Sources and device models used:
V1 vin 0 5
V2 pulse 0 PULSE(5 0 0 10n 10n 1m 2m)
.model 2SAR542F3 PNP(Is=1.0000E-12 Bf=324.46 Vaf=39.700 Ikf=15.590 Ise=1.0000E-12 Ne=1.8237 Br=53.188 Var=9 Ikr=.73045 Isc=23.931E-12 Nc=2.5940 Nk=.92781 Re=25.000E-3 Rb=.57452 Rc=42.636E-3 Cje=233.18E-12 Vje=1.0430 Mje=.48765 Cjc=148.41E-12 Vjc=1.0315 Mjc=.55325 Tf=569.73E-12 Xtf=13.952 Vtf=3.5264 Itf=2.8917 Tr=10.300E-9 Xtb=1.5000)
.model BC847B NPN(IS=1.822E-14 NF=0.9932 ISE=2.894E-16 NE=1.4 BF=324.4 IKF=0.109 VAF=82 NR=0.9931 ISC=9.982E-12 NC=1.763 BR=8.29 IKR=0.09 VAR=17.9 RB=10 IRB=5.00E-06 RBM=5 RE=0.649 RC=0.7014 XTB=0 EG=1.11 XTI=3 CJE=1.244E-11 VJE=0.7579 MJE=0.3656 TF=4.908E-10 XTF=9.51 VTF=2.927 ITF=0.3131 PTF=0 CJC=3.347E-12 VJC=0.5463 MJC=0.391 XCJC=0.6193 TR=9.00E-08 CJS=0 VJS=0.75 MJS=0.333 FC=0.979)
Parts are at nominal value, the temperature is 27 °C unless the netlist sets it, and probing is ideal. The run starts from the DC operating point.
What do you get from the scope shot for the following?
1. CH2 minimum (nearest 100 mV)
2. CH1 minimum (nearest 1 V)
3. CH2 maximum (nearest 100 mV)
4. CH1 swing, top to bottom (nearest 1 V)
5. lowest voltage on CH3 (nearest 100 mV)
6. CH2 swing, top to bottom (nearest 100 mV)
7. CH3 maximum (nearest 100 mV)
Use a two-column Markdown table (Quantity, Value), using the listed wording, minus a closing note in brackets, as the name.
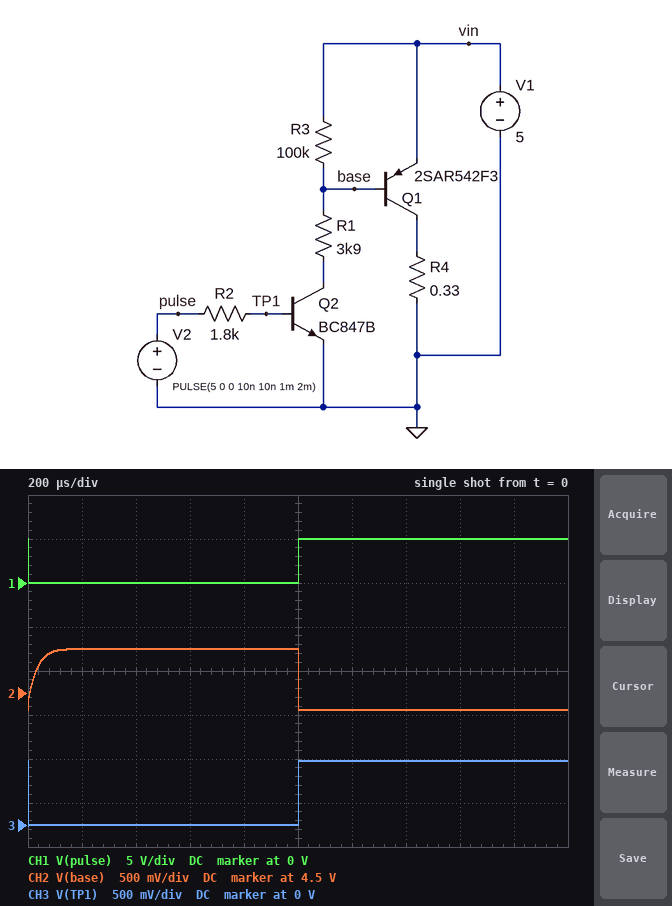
| Quantity | Value |
|---|---|
| CH2 minimum | 4.3 V |
| CH1 minimum | 0 V |
| CH2 maximum | 5.0 V |
| CH1 swing, top to bottom | 5 V |
| lowest voltage on CH3 | 0 V |
| CH2 swing, top to bottom | 700 mV |
| CH3 maximum | 700 mV |
